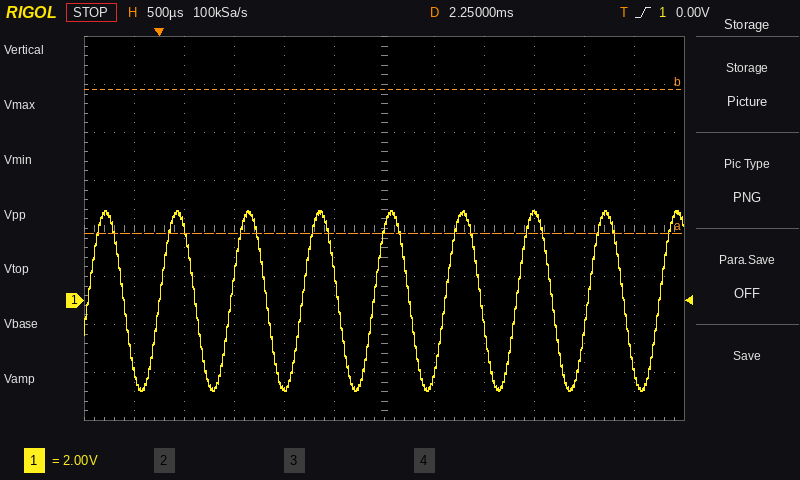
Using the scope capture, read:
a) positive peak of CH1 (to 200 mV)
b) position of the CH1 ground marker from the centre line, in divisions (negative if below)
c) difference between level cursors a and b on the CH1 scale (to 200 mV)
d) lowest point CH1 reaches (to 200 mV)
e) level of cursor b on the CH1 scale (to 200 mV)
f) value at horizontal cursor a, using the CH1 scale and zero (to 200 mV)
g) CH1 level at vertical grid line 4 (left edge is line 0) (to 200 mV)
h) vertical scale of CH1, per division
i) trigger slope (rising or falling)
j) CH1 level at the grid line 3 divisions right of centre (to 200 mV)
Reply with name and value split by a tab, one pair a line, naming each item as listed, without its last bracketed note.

positive peak of CH1	3.8 V
position of the CH1 ground marker from the centre line, in divisions	-1.5 div
difference between level cursors a and b on the CH1 scale	6.0 V
lowest point CH1 reaches	-3.8 V
level of cursor b on the CH1 scale	8.8 V
value at horizontal cursor a, using the CH1 scale and zero	2.8 V
CH1 level at vertical grid line 4 (left edge is line 0)	-3.6 V
vertical scale of CH1, per division	2 V
trigger slope	rising
CH1 level at the grid line 3 divisions right of centre	3.6 V
